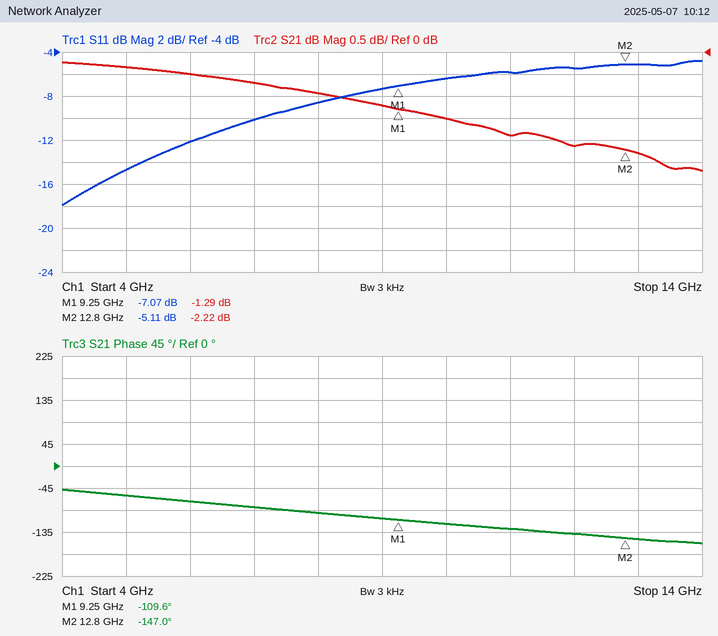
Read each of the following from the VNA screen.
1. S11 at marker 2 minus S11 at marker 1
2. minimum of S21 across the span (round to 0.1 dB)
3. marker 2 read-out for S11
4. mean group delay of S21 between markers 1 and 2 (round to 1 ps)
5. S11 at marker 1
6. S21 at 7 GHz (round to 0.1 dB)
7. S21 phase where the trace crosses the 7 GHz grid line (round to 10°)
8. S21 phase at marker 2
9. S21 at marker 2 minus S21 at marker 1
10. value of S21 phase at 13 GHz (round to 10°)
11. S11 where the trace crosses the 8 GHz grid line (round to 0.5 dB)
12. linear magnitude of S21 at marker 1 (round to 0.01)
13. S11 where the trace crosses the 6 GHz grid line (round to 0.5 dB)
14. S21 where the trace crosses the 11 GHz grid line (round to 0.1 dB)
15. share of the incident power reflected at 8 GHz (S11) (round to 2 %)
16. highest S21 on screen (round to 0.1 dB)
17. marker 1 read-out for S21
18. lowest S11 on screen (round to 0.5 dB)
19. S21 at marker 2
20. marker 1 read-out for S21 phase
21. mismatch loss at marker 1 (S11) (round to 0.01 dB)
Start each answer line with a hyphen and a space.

- 1.96 dB
- -2.7 dB
- -5.11 dB
- 29 ps
- -7.07 dB
- -0.7 dB
- -80°
- -147.0°
- -0.93 dB
- -150°
- -8.5 dB
- 0.86
- -12.0 dB
- -1.9 dB
- 14 %
- -0.2 dB
- -1.29 dB
- -18.0 dB
- -2.22 dB
- -109.6°
- 0.95 dB
